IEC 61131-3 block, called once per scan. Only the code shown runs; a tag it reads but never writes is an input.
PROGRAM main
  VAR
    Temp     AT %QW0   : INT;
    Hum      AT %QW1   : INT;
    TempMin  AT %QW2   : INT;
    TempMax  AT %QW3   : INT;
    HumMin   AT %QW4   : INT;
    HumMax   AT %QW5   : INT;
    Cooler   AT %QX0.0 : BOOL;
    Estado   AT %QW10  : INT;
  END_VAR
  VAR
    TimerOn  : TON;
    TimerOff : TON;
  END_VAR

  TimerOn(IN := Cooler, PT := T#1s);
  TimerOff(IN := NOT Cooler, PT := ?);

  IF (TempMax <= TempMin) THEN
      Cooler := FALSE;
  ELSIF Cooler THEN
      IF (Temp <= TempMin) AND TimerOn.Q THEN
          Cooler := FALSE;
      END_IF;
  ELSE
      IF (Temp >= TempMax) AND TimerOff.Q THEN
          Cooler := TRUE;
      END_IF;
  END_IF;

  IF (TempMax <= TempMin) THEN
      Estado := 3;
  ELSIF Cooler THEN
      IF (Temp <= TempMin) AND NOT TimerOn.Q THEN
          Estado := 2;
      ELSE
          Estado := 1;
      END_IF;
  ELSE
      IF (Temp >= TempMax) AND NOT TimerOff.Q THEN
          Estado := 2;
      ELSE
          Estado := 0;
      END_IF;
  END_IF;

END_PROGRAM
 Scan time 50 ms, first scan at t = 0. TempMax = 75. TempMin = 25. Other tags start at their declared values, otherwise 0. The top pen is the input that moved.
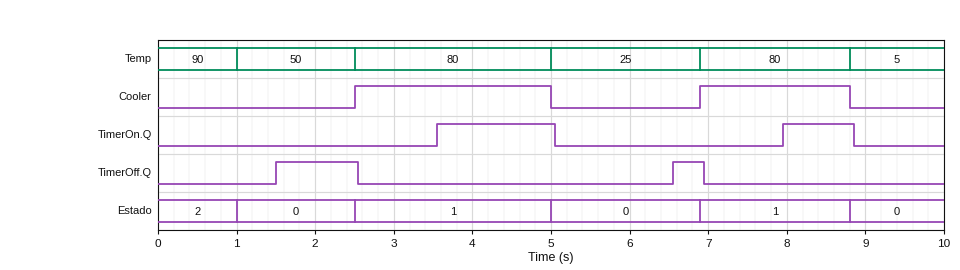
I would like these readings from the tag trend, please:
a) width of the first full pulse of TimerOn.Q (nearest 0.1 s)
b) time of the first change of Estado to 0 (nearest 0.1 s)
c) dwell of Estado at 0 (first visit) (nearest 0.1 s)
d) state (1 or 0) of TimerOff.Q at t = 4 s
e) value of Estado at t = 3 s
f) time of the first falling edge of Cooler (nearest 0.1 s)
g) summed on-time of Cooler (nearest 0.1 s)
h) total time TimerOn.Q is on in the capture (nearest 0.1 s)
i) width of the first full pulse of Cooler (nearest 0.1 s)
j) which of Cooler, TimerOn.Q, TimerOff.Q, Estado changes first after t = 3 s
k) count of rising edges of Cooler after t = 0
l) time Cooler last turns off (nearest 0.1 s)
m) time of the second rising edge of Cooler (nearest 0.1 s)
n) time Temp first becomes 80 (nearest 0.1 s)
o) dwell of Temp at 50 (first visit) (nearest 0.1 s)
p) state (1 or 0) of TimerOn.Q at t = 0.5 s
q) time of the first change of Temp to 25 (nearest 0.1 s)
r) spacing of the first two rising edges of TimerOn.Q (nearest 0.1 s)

1.5 s
1.0 s
1.5 s
0
1
5.0 s
4.4 s
2.4 s
2.5 s
TimerOn.Q
2
8.8 s
6.9 s
2.5 s
1.5 s
0
5.0 s
4.4 s
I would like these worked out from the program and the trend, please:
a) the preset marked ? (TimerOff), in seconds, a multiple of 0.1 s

1.5 s
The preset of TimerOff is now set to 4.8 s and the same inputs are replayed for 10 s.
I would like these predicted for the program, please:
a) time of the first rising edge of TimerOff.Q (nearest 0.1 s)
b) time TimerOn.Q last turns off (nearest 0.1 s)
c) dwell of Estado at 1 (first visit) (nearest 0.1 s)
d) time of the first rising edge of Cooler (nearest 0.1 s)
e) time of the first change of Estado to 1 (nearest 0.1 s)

4.8 s
5.9 s
0.2 s
4.8 s
4.8 s
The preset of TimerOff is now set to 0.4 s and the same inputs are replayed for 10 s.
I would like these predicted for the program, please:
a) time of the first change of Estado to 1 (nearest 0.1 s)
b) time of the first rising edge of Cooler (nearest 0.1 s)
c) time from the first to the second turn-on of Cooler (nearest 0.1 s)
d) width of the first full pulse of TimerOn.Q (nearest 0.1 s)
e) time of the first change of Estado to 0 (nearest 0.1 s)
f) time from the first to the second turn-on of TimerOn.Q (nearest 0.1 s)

0.4 s
0.4 s
6.5 s
3.6 s
5.0 s
6.5 s
